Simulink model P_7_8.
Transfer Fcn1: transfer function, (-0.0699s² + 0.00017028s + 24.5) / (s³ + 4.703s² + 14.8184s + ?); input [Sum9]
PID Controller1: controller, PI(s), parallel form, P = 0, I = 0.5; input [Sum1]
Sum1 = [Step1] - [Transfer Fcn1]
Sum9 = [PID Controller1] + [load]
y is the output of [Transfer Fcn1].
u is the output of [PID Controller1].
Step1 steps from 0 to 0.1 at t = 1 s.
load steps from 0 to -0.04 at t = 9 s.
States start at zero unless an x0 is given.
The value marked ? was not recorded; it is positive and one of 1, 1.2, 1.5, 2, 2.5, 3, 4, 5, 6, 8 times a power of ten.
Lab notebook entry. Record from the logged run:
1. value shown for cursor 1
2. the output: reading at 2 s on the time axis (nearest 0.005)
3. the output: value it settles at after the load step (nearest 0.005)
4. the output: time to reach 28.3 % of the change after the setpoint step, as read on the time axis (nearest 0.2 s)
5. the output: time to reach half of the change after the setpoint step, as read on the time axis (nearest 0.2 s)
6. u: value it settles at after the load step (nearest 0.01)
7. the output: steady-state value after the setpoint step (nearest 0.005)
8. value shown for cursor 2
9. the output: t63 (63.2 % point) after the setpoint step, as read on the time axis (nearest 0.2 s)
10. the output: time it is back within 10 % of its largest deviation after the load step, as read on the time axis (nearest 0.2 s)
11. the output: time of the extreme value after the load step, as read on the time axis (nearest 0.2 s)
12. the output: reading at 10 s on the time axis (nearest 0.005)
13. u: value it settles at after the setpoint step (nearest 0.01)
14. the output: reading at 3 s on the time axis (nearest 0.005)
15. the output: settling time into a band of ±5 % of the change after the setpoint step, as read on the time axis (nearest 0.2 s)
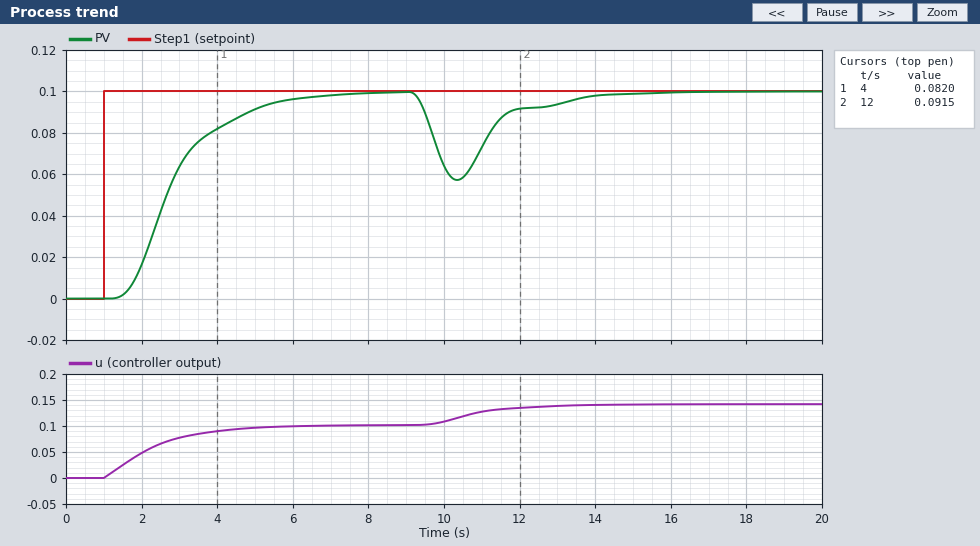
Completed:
0.0820
0.015
0.100
2.2 s
2.6 s
0.14
0.100
0.0915
3.0 s
13.4 s
10.4 s
0.065
0.10
0.065
5.6 s
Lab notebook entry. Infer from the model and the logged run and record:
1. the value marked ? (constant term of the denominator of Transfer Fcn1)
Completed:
25
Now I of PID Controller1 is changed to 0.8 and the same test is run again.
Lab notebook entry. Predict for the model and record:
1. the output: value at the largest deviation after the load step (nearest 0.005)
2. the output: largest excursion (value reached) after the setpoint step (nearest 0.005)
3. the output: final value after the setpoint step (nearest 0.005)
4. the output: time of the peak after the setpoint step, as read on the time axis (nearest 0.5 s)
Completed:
0.060
0.105
0.100
3.5 s
